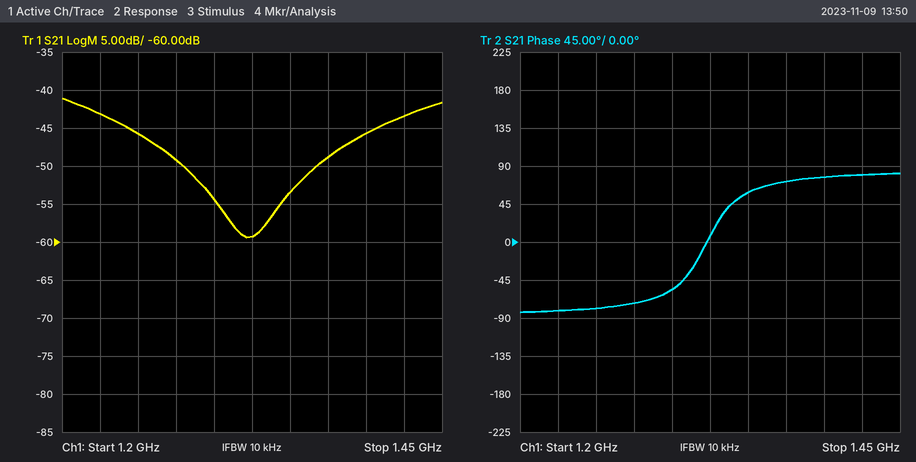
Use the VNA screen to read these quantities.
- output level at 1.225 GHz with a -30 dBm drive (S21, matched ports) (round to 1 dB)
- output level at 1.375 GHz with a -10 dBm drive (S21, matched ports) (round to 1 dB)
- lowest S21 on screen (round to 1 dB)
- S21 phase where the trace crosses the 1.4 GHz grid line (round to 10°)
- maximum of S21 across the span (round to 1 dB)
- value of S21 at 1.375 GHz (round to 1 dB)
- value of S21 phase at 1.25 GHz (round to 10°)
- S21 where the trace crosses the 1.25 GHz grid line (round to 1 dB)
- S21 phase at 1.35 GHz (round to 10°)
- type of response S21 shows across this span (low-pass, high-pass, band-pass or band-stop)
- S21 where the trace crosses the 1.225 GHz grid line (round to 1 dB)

-73 dBm
-59 dBm
-59 dB
80°
-41 dB
-49 dB
-80°
-46 dB
60°
band-stop
-43 dB
